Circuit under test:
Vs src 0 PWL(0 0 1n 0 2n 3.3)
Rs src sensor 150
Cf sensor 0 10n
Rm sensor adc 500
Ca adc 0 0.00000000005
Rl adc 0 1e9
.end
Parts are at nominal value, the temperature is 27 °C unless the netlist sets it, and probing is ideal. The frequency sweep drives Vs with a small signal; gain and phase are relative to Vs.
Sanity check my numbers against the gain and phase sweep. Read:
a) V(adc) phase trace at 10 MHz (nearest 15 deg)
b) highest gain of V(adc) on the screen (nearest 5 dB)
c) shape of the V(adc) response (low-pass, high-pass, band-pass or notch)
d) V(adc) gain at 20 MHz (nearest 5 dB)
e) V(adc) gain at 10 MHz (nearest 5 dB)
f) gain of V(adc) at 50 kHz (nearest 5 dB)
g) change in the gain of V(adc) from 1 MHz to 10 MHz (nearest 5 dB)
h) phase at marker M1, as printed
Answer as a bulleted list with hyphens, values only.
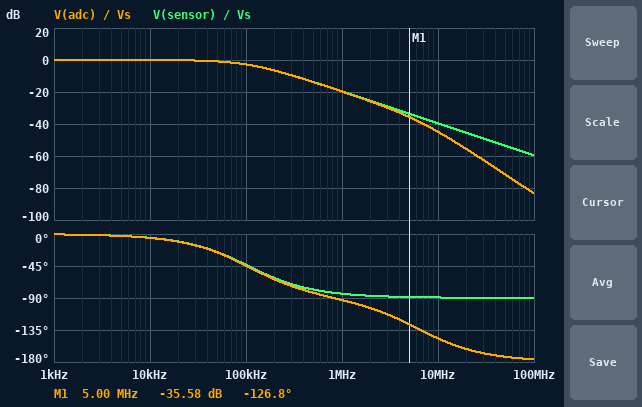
- -150 deg
- 0 dB
- low-pass
- -55 dB
- -45 dB
- 0 dB
- -25 dB
- -126.8 deg
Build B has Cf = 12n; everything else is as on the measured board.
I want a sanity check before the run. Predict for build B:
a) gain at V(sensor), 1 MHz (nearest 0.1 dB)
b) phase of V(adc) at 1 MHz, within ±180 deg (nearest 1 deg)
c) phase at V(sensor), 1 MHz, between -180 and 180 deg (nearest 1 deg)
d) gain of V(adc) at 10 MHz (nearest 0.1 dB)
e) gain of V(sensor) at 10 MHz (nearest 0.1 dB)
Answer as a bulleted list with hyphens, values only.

- -21.1 dB
- -94 deg
- -85 deg
- -46.5 dB
- -41.1 dB
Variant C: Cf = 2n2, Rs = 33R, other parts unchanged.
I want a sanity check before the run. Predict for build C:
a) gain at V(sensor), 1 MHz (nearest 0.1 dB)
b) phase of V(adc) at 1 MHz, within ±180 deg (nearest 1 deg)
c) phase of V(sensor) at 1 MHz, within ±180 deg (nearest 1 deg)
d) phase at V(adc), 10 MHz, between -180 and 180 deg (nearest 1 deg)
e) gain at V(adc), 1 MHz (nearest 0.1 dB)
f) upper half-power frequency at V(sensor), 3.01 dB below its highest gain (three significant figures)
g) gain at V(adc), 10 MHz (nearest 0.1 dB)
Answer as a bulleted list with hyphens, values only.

- -0.9 dB
- -34 deg
- -25 deg
- -135 deg
- -1.0 dB
- 2.13 MHz
- -18.9 dB
